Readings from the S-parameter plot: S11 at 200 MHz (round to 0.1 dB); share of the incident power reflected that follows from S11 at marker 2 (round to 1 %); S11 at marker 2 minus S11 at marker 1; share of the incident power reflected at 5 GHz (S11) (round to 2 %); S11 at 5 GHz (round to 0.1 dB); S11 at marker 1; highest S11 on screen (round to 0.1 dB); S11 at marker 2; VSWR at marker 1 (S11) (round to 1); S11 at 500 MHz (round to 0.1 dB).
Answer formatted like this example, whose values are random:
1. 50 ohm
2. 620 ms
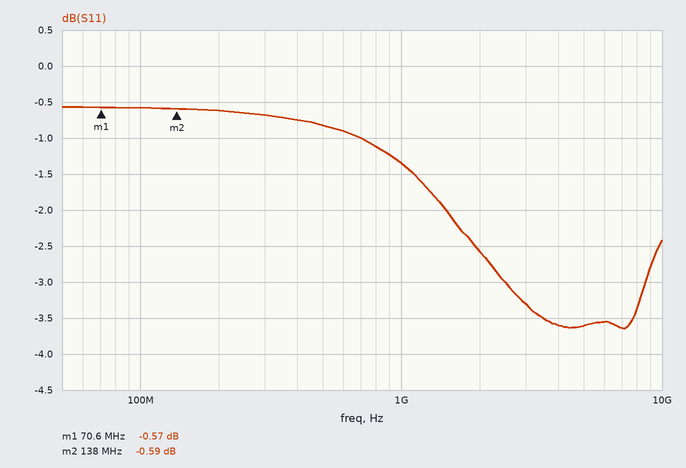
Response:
1. -0.6 dB
2. 87 %
3. -0.02 dB
4. 44 %
5. -3.6 dB
6. -0.57 dB
7. -0.6 dB
8. -0.59 dB
9. 30
10. -0.8 dB
